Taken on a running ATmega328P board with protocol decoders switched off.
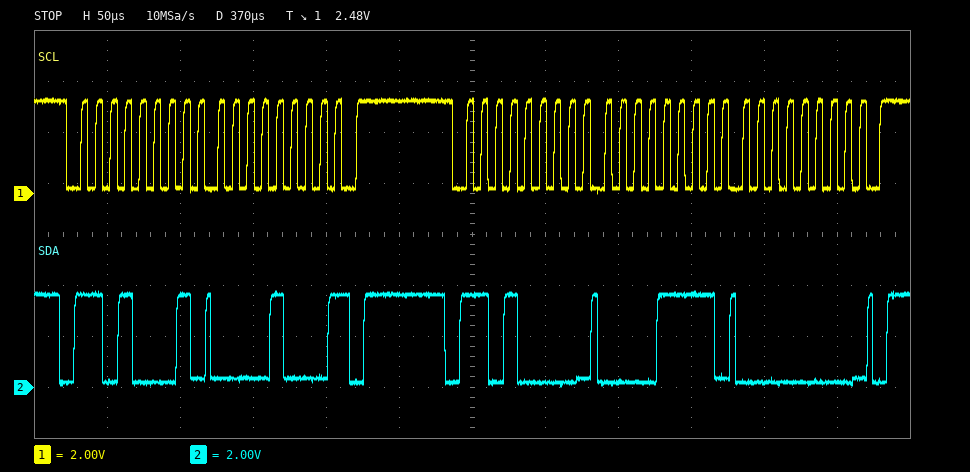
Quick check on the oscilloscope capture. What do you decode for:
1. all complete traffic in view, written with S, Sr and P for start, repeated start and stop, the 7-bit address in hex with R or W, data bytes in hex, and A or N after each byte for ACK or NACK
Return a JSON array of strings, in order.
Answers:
["S 68R A 08 N P S 68W A 0F A 00 A P"]
